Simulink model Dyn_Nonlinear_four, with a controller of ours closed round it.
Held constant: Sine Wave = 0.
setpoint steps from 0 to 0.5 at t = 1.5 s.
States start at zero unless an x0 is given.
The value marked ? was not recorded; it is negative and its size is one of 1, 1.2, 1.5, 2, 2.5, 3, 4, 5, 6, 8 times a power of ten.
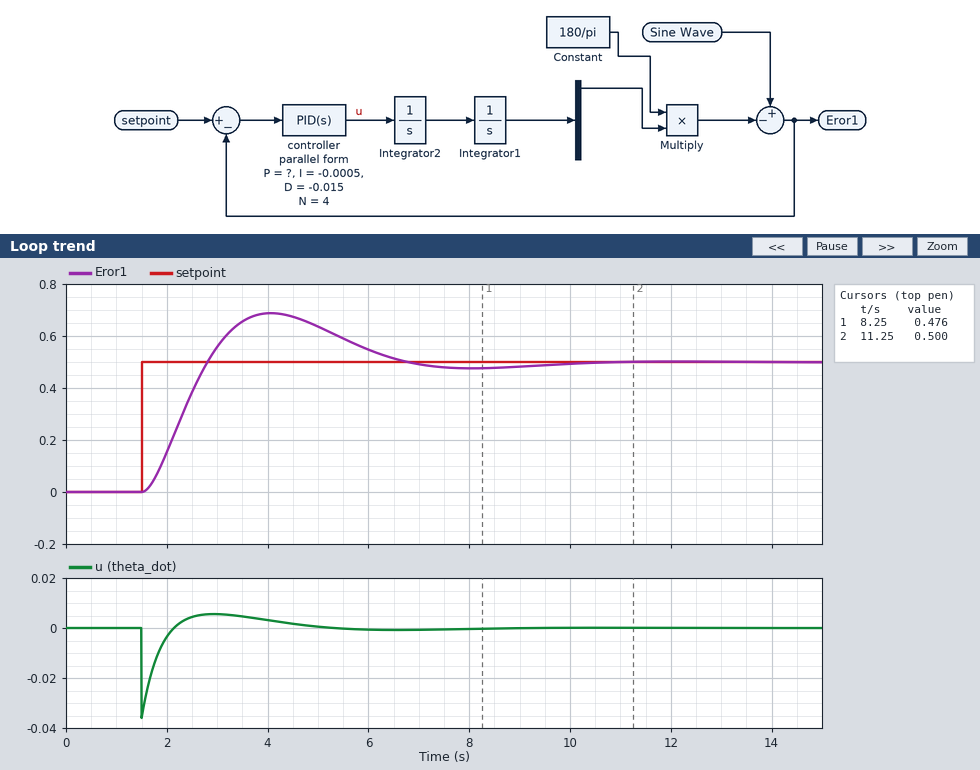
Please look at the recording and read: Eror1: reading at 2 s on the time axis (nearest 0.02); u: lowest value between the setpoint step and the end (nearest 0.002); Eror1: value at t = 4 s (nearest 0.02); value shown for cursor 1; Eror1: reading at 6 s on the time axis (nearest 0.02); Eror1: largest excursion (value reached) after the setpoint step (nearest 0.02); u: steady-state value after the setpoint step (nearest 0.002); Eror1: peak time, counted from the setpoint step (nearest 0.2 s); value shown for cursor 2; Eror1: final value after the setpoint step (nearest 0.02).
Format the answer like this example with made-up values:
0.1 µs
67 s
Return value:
0.16
-0.036
0.68
0.476
0.54
0.68
0.000
2.6 s
0.500
0.50
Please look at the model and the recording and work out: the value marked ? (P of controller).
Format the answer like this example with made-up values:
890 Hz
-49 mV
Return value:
-0.012
